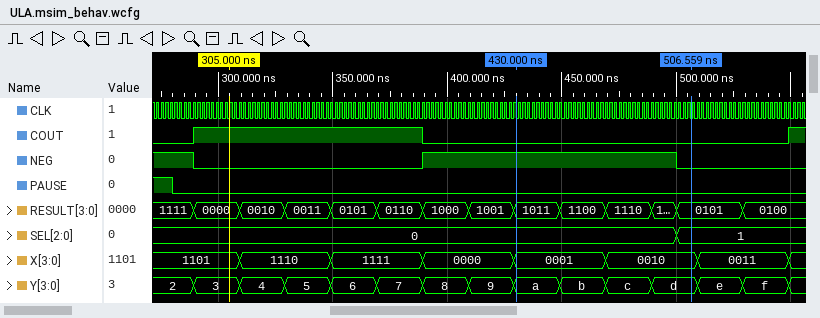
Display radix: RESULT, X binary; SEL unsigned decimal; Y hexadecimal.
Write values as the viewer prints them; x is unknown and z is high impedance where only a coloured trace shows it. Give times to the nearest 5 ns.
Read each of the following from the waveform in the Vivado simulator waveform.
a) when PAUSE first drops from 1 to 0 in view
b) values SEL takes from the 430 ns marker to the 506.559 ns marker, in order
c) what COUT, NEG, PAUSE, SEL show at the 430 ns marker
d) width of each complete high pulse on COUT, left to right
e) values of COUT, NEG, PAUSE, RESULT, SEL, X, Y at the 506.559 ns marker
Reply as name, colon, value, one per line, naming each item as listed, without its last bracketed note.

when PAUSE first drops from 1 to 0 in view: 280 ns
values SEL takes from the 430 ns marker to the 506.559 ns marker, in order: 0, 1
what COUT, NEG, PAUSE, SEL show at the 430 ns marker: COUT=0, NEG=1, PAUSE=0, SEL=0
width of each complete high pulse on COUT, left to right: 100 ns
values of COUT, NEG, PAUSE, RESULT, SEL, X, Y at the 506.559 ns marker: COUT=0, NEG=0, PAUSE=0, RESULT=0101, SEL=1, X=0010, Y=d
